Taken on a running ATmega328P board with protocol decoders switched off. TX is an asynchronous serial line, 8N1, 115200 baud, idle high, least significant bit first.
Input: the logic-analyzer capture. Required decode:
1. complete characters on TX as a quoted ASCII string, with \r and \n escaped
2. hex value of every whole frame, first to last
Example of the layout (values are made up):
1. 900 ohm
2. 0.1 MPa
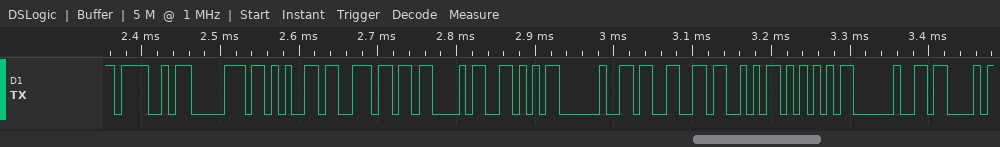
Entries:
1. "OpenCV 3SU C"
2. 0x4F 0x70 0x65 0x6E 0x43 0x56 0x20 0x33 0x53 0x55 0x20 0x43
